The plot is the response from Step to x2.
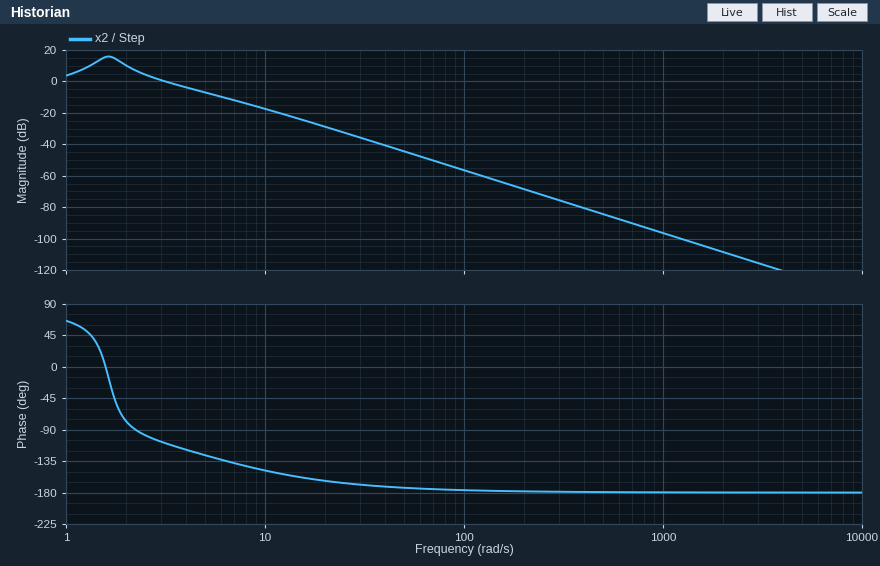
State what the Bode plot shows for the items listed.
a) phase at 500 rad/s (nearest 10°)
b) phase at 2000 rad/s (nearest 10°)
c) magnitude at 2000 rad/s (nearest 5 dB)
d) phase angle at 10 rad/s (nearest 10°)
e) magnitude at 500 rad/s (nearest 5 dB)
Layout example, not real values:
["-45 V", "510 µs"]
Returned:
["-180°", "-180°", "-110 dB", "-150°", "-85 dB"]
